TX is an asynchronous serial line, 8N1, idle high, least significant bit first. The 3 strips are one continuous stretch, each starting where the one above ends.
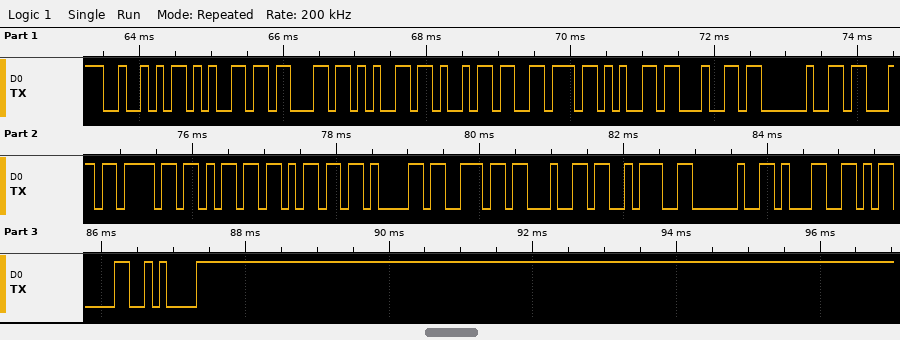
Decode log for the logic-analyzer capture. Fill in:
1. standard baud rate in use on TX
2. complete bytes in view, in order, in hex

9600 baud
0x52 0x65 0x63 0x65 0x69 0x76 0x65 0x64 0x20 0x63 0x6F 0x6D 0x6D 0x61 0x6E 0x64 0x3A 0x20 0x31 0x0D 0x0A
